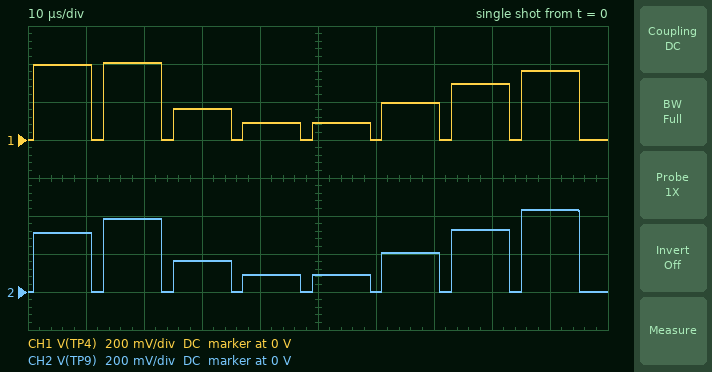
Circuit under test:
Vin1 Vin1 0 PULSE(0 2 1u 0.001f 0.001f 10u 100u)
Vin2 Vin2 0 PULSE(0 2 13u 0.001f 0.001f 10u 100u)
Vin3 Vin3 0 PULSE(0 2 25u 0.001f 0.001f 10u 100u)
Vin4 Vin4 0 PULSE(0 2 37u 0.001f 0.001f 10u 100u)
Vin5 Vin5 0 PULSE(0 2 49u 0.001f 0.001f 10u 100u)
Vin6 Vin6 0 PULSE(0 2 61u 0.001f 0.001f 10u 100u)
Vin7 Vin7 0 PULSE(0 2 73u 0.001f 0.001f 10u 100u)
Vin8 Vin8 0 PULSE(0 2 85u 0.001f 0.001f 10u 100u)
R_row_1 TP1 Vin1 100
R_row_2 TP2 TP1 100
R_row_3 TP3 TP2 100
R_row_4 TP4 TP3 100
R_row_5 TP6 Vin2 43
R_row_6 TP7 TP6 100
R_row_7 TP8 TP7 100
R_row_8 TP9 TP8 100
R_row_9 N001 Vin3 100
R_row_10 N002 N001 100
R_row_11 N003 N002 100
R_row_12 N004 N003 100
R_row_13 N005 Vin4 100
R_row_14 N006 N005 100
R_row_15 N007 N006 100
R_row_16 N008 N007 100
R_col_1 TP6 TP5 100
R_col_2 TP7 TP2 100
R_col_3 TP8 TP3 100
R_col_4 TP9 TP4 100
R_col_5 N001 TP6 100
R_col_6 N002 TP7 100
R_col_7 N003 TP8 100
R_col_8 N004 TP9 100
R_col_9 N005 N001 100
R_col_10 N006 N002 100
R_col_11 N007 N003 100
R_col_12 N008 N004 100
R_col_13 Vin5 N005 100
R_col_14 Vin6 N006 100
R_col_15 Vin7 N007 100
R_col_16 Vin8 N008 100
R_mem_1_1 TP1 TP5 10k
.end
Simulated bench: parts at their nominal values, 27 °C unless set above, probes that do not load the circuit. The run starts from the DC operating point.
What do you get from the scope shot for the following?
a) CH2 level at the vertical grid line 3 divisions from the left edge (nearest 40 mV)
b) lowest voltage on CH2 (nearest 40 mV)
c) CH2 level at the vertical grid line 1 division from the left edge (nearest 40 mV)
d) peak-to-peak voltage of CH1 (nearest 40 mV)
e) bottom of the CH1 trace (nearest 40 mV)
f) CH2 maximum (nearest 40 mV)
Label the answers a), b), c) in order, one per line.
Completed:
a) 160 mV
b) 0 V
c) 320 mV
d) 400 mV
e) 0 V
f) 440 mV
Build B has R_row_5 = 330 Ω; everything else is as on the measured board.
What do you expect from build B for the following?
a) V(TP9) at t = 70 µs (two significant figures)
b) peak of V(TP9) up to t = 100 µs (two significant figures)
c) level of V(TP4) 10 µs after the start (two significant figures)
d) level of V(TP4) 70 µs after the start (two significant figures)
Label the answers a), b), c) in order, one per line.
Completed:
a) 240 mV
b) 460 mV
c) 440 mV
d) 230 mV
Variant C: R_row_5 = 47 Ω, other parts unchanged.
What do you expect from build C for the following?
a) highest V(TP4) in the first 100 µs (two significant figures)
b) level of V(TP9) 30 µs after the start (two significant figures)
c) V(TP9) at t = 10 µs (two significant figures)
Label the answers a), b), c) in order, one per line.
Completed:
a) 400 mV
b) 170 mV
c) 310 mV
